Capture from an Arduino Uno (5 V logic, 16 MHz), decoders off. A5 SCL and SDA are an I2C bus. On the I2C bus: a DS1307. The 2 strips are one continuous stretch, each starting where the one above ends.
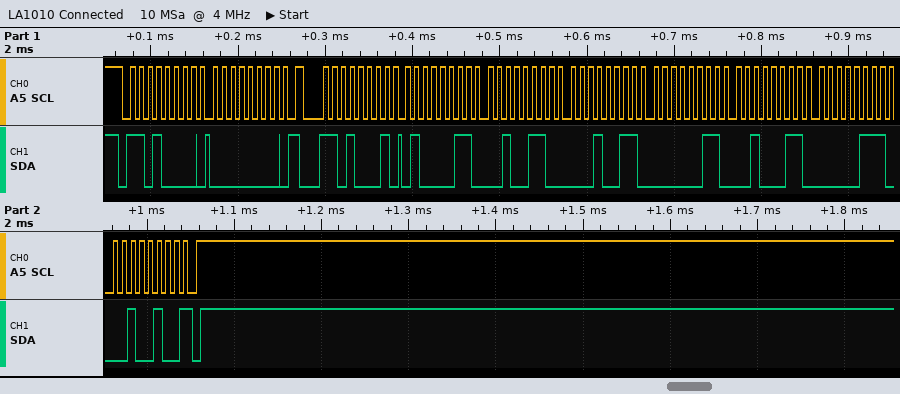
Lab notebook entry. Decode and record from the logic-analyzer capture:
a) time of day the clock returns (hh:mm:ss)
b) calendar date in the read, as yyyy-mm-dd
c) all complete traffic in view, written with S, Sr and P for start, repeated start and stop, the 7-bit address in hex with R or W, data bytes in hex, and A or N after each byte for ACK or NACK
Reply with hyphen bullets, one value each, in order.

- 13:26:43
- 2024-07-23
- S 68W A 00 A Sr 68R A 43 A 26 A 13 A 03 A 23 A 07 A 24 N P
